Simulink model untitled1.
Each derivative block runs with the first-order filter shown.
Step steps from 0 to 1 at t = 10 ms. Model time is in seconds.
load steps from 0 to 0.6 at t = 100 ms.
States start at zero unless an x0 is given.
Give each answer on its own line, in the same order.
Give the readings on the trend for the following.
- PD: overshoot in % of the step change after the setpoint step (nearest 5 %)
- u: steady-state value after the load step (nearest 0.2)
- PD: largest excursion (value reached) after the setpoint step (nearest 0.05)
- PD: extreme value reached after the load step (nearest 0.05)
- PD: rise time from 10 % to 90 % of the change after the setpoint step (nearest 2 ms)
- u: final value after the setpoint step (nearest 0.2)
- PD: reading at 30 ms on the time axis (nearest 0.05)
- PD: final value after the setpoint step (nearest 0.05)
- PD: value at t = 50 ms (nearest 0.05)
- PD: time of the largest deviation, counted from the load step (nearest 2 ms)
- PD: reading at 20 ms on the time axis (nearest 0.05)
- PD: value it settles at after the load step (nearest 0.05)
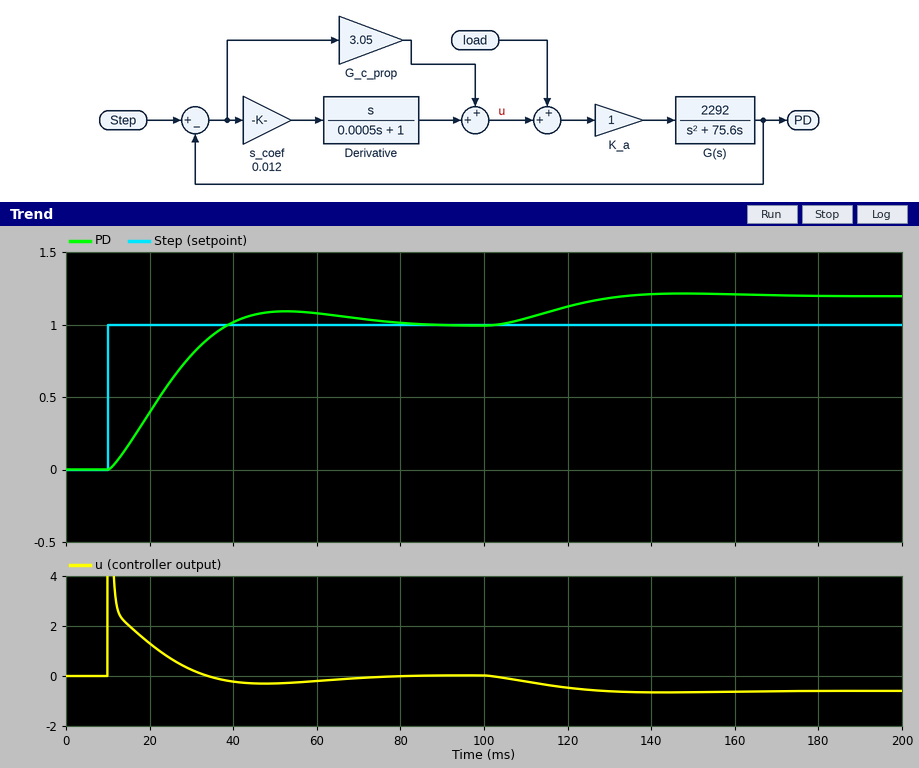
10 %
-0.6
1.10
1.20
20 ms
0.0
0.80
1.00
1.10
48 ms
0.40
1.20
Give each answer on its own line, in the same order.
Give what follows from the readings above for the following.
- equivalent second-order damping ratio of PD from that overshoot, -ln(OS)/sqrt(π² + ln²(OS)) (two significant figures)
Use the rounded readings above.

0.59
